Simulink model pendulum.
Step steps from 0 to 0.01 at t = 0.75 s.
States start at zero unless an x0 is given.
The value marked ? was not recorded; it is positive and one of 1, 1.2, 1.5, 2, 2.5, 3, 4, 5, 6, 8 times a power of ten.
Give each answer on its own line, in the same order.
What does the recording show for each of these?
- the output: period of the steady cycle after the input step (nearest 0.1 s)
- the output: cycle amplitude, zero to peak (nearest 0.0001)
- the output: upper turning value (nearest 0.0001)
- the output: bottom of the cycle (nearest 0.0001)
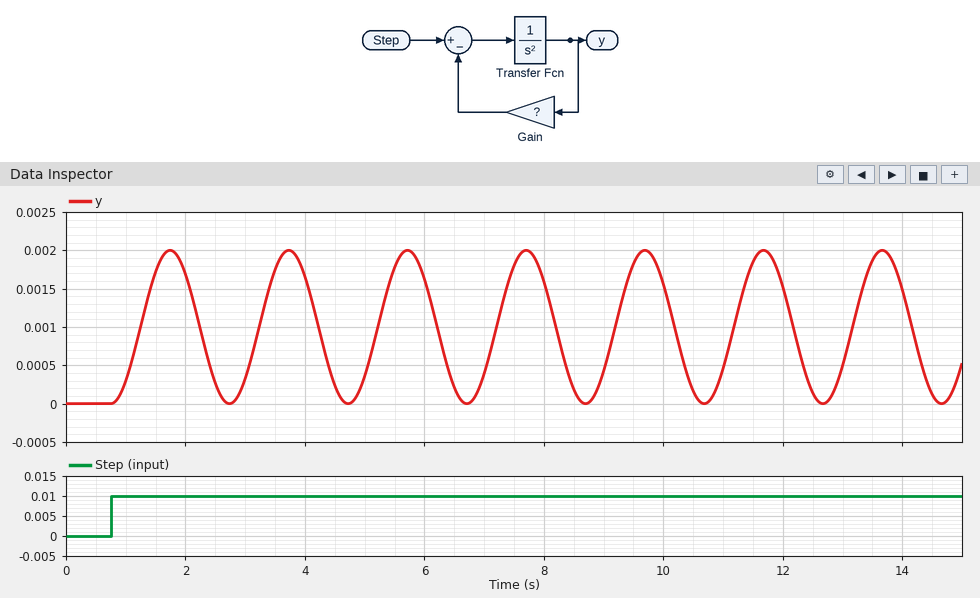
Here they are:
2.0 s
0.0010
0.0020
0.0000
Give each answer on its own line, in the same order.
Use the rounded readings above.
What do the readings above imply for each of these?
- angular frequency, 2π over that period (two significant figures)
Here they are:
3.1 rad/s
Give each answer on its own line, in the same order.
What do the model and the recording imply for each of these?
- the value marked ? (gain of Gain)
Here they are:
10
